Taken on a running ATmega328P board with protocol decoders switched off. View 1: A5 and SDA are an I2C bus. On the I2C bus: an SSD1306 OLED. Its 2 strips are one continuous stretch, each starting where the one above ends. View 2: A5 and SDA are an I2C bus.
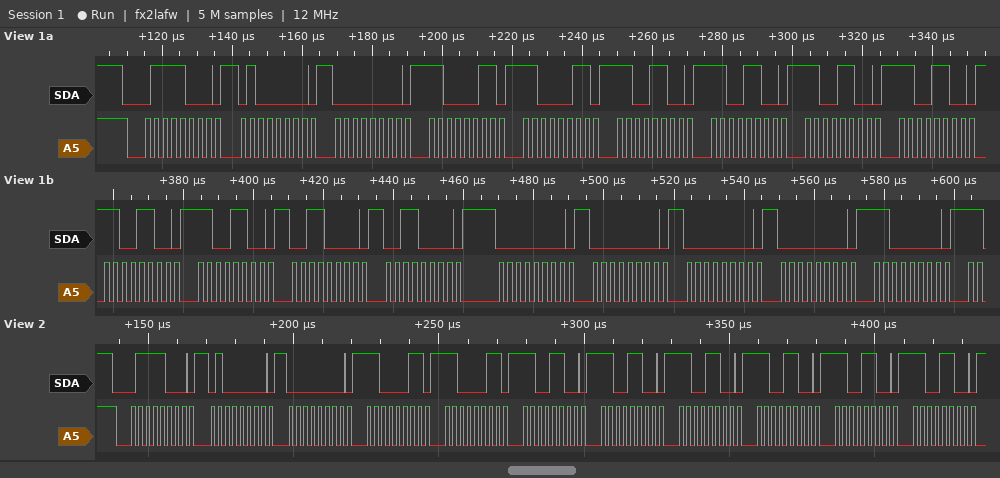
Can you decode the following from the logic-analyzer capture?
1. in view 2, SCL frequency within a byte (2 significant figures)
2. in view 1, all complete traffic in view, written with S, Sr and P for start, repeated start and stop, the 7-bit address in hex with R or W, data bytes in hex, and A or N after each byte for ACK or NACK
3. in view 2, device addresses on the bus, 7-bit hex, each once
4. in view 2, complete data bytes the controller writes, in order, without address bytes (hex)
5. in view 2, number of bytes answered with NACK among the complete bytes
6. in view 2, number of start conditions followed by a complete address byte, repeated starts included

400 kHz
S 3CW A 40 A 00 A C3 A C3 A CC A CC A CC A CC A CC A CC A 30 A 30 A 00 A 00 A 00 A 00 A C0 A
0x3C
40 00 C3 C3 CC CC CC CC CC CC
0
1
